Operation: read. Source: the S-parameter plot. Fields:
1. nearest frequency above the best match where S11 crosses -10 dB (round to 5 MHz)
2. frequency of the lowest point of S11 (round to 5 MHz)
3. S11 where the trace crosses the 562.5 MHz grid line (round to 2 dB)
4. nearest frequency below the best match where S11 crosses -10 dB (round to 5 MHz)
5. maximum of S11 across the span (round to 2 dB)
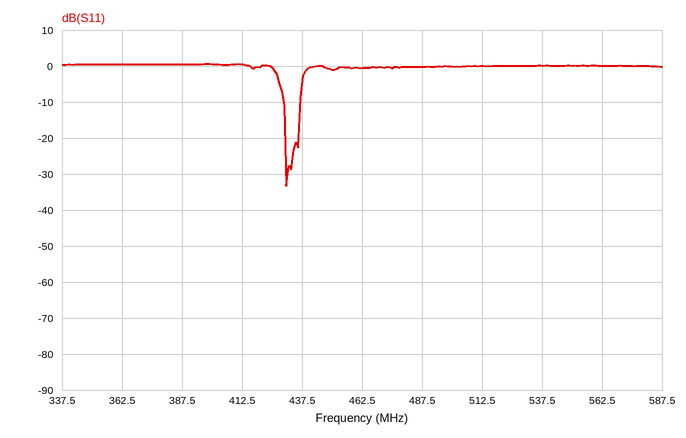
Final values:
435 MHz
430 MHz
0 dB
430 MHz
0 dB
